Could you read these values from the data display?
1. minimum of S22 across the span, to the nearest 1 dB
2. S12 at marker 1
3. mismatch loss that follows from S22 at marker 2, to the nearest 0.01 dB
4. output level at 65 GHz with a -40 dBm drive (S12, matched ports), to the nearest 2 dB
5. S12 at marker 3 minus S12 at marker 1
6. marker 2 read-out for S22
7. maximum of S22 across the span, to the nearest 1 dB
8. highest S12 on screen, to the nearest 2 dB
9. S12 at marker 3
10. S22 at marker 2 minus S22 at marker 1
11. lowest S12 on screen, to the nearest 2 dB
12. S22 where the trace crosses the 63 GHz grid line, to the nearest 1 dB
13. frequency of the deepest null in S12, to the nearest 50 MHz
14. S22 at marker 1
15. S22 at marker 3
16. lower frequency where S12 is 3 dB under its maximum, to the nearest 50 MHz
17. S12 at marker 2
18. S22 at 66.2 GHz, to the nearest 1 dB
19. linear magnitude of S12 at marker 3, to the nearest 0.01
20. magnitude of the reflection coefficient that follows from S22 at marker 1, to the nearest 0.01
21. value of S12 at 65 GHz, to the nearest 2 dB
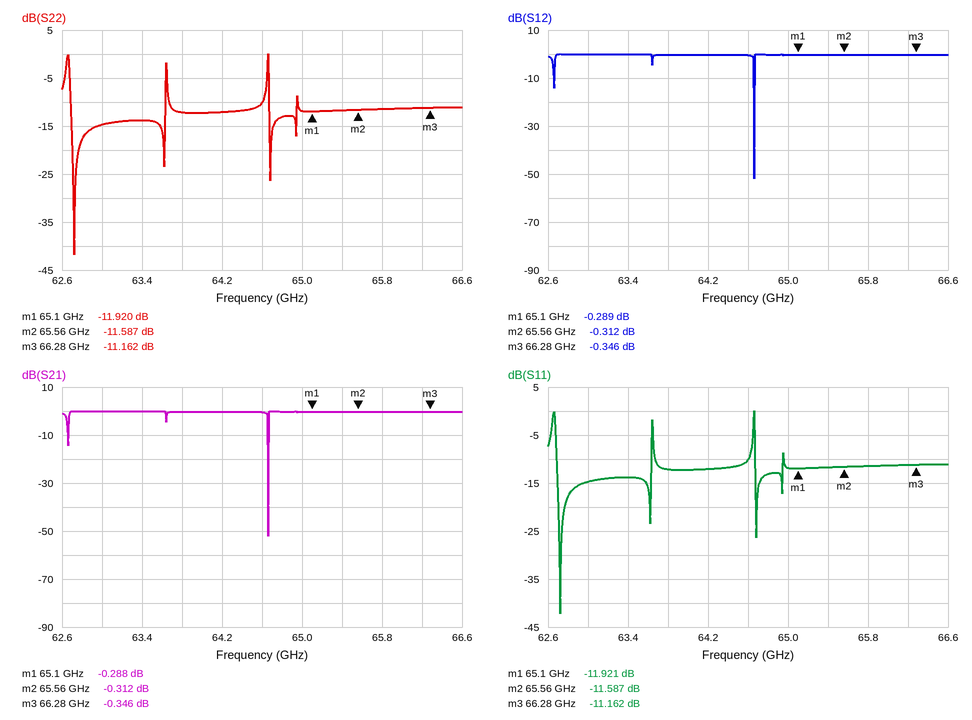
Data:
-42 dB
-0.289 dB
0.31 dB
-40 dBm
-0.057 dB
-11.587 dB
0 dB
0 dB
-0.346 dB
0.333 dB
-52 dB
-15 dB
64.65 GHz
-11.920 dB
-11.162 dB
62.65 GHz
-0.312 dB
-11 dB
0.96
0.25
0 dB
